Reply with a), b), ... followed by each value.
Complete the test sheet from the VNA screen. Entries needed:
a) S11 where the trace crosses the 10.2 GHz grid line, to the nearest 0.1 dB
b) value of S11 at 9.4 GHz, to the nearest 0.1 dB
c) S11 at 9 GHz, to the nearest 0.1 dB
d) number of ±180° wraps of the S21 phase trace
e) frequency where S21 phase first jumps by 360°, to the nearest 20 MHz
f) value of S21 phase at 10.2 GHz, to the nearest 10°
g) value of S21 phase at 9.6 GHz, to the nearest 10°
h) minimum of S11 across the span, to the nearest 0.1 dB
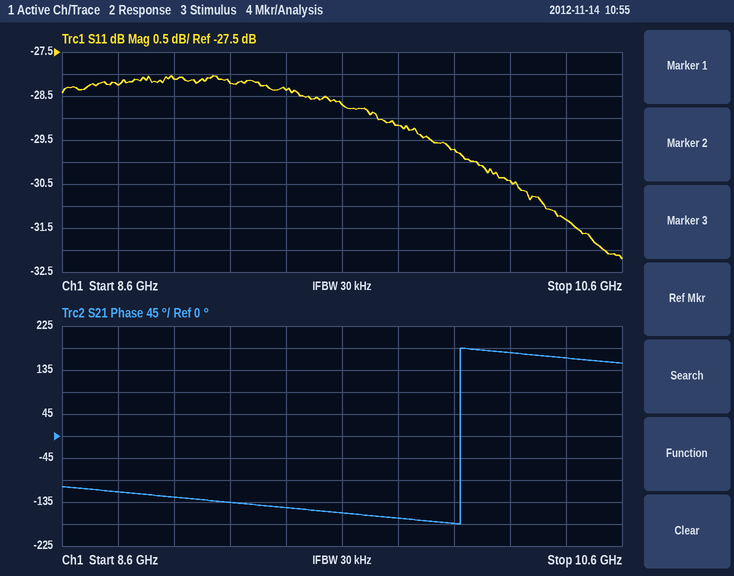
a) -30.4 dB
b) -28.4 dB
c) -28.1 dB
d) 1
e) 10.02 GHz
f) 170°
g) -160°
h) -32.2 dB
